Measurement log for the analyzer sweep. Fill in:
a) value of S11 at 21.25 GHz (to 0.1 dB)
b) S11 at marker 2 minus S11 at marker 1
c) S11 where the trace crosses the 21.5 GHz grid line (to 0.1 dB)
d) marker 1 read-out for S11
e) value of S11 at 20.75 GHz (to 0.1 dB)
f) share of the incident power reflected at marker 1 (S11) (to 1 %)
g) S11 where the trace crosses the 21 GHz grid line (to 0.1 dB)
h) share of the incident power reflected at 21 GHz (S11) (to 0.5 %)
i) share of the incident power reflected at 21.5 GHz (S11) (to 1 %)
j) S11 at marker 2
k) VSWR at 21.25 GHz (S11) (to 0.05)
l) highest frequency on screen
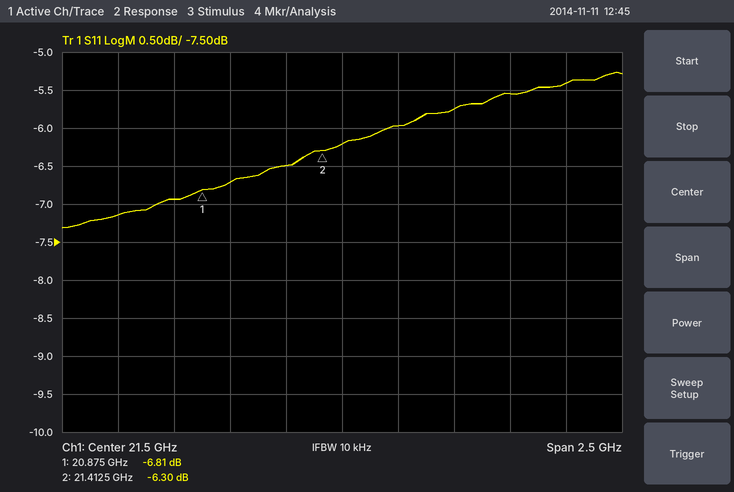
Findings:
-6.5 dB
0.51 dB
-6.2 dB
-6.81 dB
-6.9 dB
21 %
-6.7 dB
21.5 %
24 %
-6.30 dB
2.80
22.75 GHz
